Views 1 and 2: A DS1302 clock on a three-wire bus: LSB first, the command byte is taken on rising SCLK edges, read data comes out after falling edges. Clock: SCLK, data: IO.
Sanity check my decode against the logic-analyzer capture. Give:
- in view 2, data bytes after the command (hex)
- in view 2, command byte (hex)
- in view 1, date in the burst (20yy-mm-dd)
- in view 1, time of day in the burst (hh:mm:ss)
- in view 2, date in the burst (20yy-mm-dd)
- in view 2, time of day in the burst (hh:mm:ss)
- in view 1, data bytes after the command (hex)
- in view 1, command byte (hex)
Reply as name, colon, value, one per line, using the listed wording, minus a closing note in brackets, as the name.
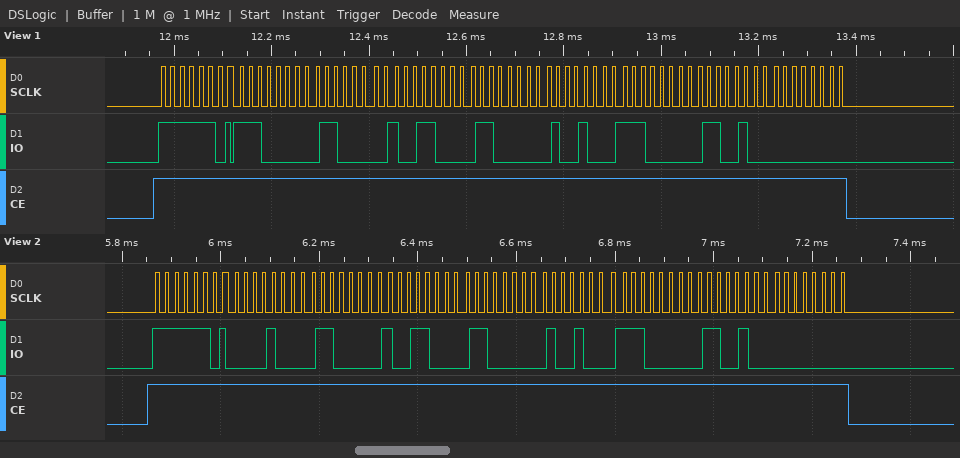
in view 2, data bytes after the command: 10 06 19 06 12 07 26 00
in view 2, command byte: 0xBF
in view 1, date in the burst: 2026-12-06
in view 1, time of day in the burst: 19:06:07
in view 2, date in the burst: 2026-12-06
in view 2, time of day in the burst: 19:06:10
in view 1, data bytes after the command: 07 06 19 06 12 07 26 00
in view 1, command byte: 0xBF
